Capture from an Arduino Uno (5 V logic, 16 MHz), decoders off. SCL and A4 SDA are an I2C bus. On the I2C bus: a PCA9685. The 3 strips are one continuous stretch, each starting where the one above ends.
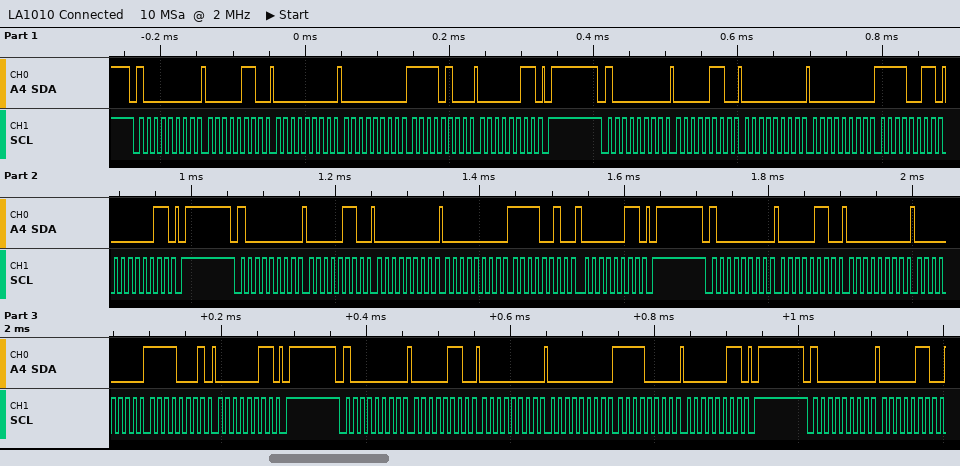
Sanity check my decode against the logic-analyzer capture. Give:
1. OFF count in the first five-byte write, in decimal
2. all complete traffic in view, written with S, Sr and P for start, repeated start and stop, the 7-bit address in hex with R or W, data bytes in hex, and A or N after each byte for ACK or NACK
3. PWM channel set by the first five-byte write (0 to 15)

1012
S 40W A 06 A 00 A 00 A F4 A 03 A P S 40W A 06 A 00 A 00 A F3 A 03 A P S 40W A 06 A 00 A 00 A F2 A 03 A P S 40W A 06 A 00 A 00 A F1 A 03 A P S 40W A 06 A 00 A 00 A F0 A 03 A P S 40W A 06 A
0
